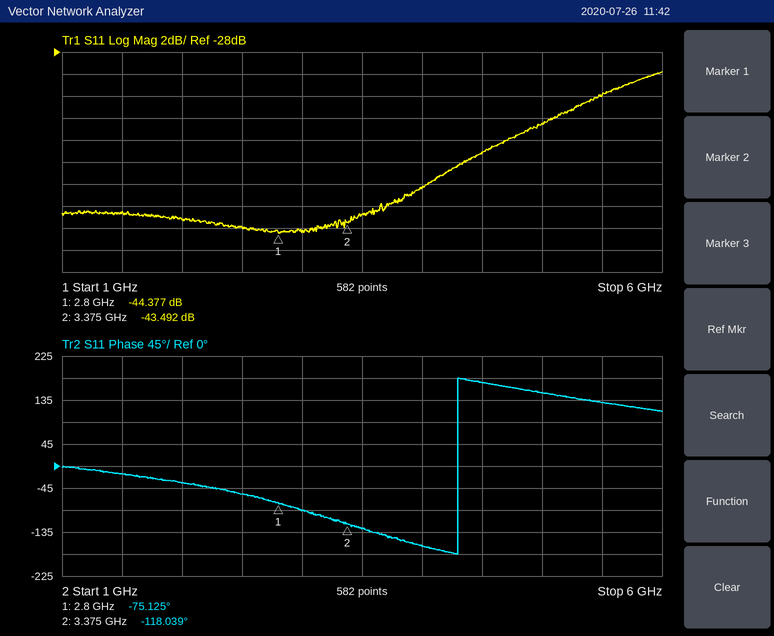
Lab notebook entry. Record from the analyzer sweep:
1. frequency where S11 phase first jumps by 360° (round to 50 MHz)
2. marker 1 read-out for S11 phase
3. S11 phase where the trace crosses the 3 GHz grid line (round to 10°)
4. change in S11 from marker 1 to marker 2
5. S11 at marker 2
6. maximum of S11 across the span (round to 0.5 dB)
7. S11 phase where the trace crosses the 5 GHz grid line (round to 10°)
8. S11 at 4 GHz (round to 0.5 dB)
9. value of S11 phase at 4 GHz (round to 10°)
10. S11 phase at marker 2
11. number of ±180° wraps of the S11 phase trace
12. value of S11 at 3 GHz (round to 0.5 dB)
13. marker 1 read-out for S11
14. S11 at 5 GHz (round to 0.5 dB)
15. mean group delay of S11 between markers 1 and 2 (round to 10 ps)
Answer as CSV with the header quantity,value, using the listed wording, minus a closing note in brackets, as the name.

quantity,value
frequency where S11 phase first jumps by 360°,4.30 GHz
marker 1 read-out for S11 phase,-75.125°
S11 phase where the trace crosses the 3 GHz grid line,-90°
change in S11 from marker 1 to marker 2,0.885 dB
S11 at marker 2,-43.492 dB
maximum of S11 across the span,-30.0 dB
S11 phase where the trace crosses the 5 GHz grid line,150°
S11 at 4 GHz,-40.5 dB
value of S11 phase at 4 GHz,-160°
S11 phase at marker 2,-118.039°
number of ±180° wraps of the S11 phase trace,1
value of S11 at 3 GHz,-44.5 dB
marker 1 read-out for S11,-44.377 dB
S11 at 5 GHz,-34.5 dB
mean group delay of S11 between markers 1 and 2,210 ps
